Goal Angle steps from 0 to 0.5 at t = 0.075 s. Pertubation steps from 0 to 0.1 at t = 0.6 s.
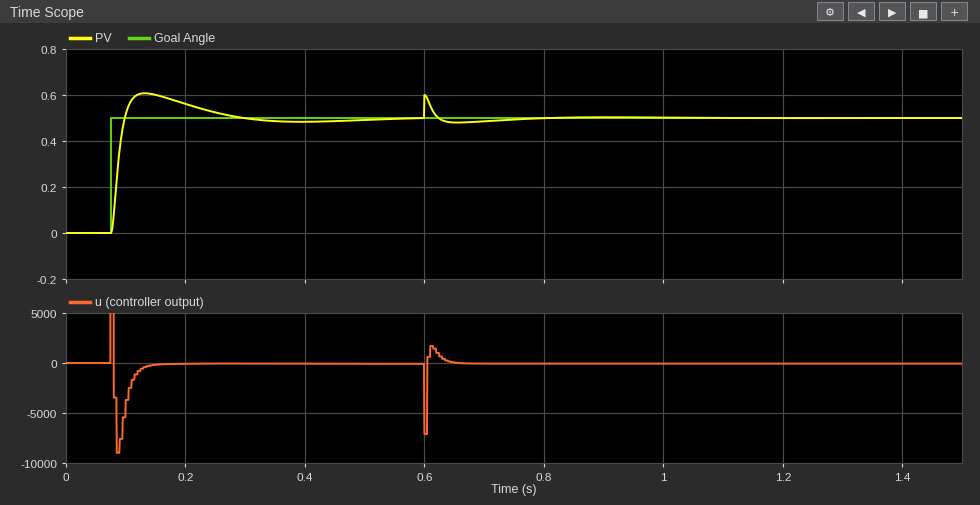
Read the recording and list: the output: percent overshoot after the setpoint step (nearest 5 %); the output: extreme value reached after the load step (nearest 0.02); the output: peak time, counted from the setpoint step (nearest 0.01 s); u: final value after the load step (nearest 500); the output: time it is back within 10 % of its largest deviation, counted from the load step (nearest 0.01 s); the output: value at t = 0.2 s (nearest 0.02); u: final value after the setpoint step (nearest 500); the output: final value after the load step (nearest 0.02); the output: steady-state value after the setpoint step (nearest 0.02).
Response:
20 %
0.60
0.06 s
0
0.13 s
0.56
0
0.50
0.50
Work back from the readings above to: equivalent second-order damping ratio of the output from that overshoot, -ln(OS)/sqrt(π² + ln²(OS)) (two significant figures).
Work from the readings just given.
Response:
0.46
